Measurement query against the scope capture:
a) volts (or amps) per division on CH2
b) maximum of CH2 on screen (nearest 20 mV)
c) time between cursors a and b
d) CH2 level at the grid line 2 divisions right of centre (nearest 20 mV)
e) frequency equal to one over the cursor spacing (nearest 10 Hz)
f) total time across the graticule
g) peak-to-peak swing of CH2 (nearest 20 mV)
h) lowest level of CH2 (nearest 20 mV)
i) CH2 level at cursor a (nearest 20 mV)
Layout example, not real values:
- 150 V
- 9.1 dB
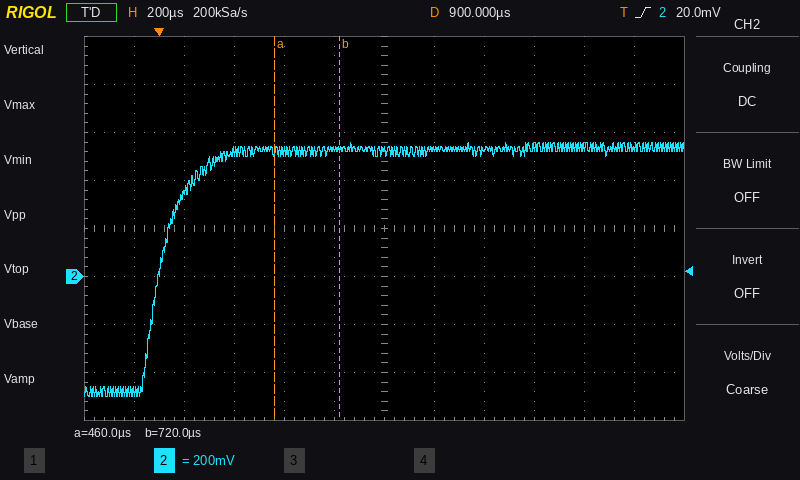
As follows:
- 200 mV
- 560 mV
- 260 µs
- 520 mV
- 3.85 kHz
- 2.4 ms
- 1.06 V
- -500 mV
- 520 mV
